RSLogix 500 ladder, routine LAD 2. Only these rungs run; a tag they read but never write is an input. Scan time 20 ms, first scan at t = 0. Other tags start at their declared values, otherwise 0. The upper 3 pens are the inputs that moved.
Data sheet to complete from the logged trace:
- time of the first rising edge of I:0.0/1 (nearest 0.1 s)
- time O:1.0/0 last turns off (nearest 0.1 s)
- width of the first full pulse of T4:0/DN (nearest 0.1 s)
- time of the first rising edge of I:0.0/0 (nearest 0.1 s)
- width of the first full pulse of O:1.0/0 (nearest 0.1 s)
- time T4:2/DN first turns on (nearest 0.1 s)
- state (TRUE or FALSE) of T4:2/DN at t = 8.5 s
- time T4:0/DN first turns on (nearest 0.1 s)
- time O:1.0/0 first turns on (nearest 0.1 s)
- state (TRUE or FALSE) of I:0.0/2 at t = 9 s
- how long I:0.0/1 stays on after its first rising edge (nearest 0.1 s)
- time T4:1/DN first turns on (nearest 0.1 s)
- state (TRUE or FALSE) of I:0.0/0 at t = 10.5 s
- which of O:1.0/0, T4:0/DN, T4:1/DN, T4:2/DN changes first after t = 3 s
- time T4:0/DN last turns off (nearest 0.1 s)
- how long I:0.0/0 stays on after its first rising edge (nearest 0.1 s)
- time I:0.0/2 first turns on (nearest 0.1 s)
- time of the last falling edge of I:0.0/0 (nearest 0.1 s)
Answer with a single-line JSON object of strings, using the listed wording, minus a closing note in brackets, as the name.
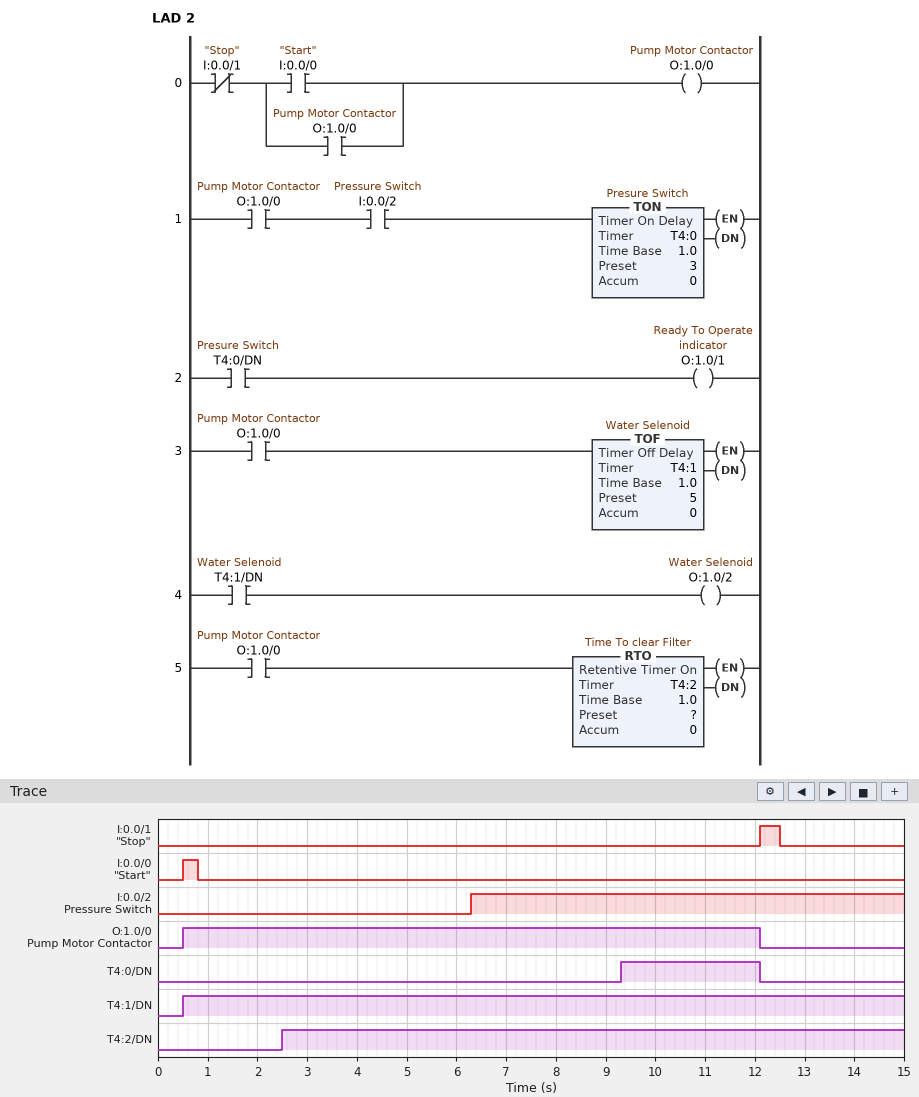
{"time of the first rising edge of I:0.0/1": "12.1 s", "time O:1.0/0 last turns off": "12.1 s", "width of the first full pulse of T4:0/DN": "2.8 s", "time of the first rising edge of I:0.0/0": "0.5 s", "width of the first full pulse of O:1.0/0": "11.6 s", "time T4:2/DN first turns on": "2.5 s", "state (TRUE or FALSE) of T4:2/DN at t = 8.5 s": "TRUE", "time T4:0/DN first turns on": "9.3 s", "time O:1.0/0 first turns on": "0.5 s", "state (TRUE or FALSE) of I:0.0/2 at t = 9 s": "TRUE", "how long I:0.0/1 stays on after its first rising edge": "0.4 s", "time T4:1/DN first turns on": "0.5 s", "state (TRUE or FALSE) of I:0.0/0 at t = 10.5 s": "FALSE", "which of O:1.0/0, T4:0/DN, T4:1/DN, T4:2/DN changes first after t = 3 s": "T4:0/DN", "time T4:0/DN last turns off": "12.1 s", "how long I:0.0/0 stays on after its first rising edge": "0.3 s", "time I:0.0/2 first turns on": "6.3 s", "time of the last falling edge of I:0.0/0": "0.8 s"}
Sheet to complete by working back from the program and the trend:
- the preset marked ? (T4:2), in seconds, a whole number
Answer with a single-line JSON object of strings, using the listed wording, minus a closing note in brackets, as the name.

{"the preset marked ? (T4:2), in seconds, a whole number": "2 s"}
